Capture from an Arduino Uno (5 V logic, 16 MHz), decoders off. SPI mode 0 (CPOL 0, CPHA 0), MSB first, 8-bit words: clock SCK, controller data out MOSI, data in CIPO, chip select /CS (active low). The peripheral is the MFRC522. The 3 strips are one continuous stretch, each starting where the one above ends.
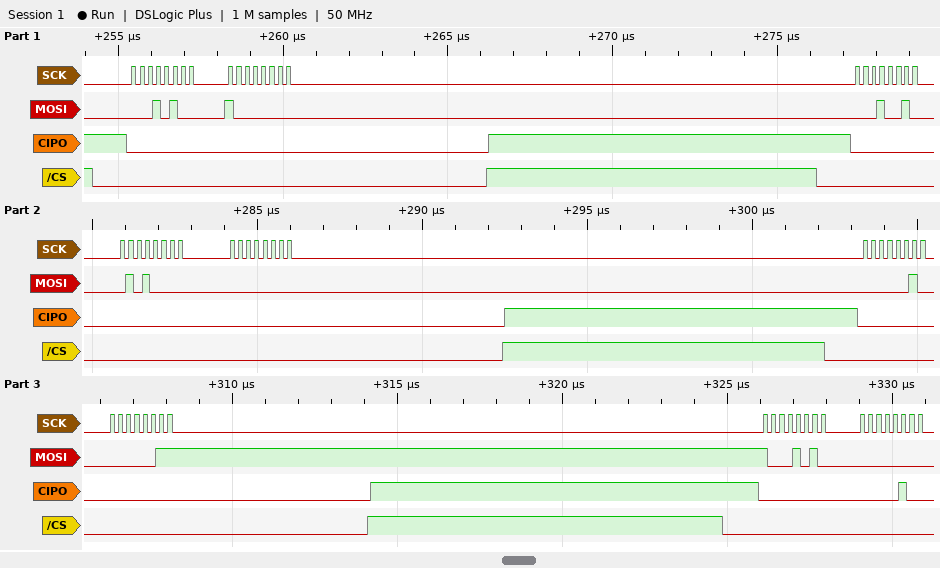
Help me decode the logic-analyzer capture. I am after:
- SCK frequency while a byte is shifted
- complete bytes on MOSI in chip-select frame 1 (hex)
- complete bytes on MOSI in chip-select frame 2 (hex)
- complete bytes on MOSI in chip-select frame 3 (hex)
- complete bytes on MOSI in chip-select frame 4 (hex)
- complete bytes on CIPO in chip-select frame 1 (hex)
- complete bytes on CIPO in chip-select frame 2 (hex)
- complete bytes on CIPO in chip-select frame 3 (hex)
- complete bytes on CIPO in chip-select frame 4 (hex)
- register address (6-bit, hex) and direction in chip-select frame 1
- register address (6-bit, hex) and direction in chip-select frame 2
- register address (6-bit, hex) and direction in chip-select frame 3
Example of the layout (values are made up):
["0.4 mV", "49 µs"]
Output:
["4 MHz", "0x14 0x80", "0x12 0x50 0x00", "0x02 0x03", "0x8A 0x00", "0x00 0x00", "0x00 0x00 0x00", "0x00 0x00", "0x00 0x04", "0x0A write", "0x09 write", "0x01 write"]
